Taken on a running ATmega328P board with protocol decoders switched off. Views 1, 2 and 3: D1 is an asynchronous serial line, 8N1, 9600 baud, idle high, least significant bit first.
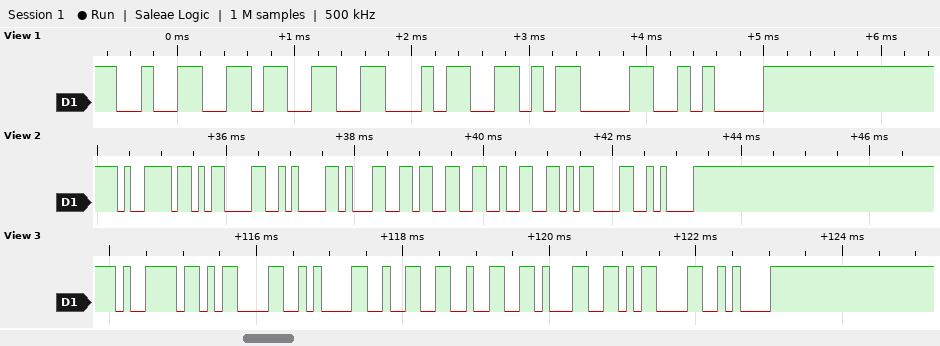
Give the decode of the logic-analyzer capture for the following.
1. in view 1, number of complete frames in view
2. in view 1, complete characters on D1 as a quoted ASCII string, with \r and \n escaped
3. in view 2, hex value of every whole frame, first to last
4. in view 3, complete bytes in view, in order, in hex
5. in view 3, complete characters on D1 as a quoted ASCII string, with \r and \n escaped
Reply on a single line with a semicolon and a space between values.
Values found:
5; "234\r\n"; 79 0D 0A 31 33 32 0D 0A; 0x79 0x0D 0x0A 0x32 0x32 0x31 0x0D 0x0A; "y\r\n221\r\n"
